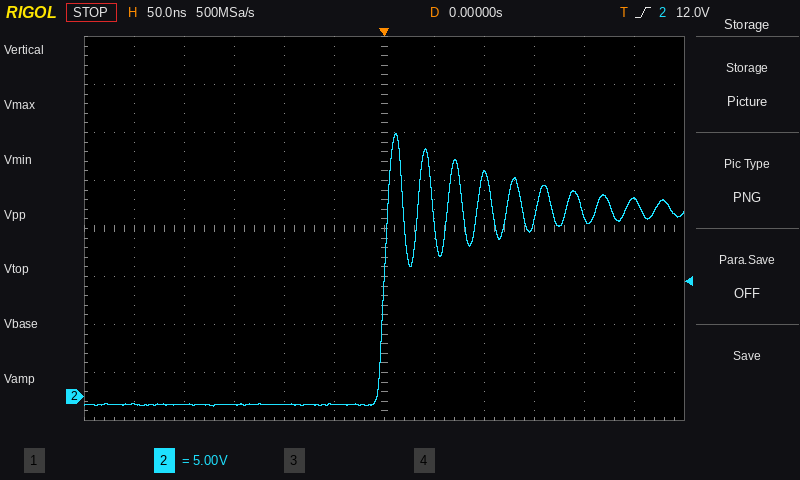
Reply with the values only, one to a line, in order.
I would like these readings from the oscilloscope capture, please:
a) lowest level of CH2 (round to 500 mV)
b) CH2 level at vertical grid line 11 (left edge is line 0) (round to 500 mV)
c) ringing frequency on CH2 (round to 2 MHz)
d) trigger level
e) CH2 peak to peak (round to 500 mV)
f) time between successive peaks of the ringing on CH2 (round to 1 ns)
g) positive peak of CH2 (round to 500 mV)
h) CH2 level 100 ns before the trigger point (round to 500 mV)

-1.0 V
20.5 V
34 MHz
12.0 V
28.5 V
30 ns
27.5 V
-1.0 V
